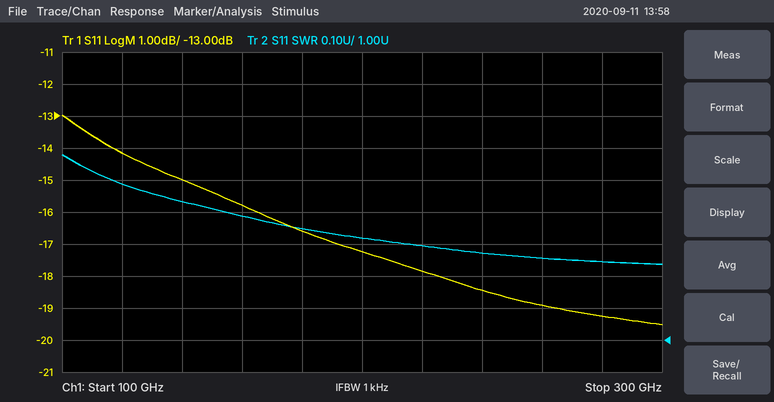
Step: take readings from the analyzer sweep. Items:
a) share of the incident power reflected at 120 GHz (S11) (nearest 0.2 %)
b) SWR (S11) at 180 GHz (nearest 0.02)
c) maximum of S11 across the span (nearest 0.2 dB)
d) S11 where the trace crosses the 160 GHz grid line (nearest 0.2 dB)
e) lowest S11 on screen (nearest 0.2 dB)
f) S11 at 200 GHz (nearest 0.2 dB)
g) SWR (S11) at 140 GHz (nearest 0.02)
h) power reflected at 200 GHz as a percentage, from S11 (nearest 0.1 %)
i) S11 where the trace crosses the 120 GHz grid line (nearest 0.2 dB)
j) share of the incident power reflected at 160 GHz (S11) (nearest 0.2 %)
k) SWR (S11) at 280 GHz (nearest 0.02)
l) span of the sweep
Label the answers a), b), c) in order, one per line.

a) 3.8 %
b) 1.34
c) -13.0 dB
d) -15.8 dB
e) -19.6 dB
f) -17.2 dB
g) 1.44
h) 1.9 %
i) -14.2 dB
j) 2.6 %
k) 1.24
l) 200 GHz
